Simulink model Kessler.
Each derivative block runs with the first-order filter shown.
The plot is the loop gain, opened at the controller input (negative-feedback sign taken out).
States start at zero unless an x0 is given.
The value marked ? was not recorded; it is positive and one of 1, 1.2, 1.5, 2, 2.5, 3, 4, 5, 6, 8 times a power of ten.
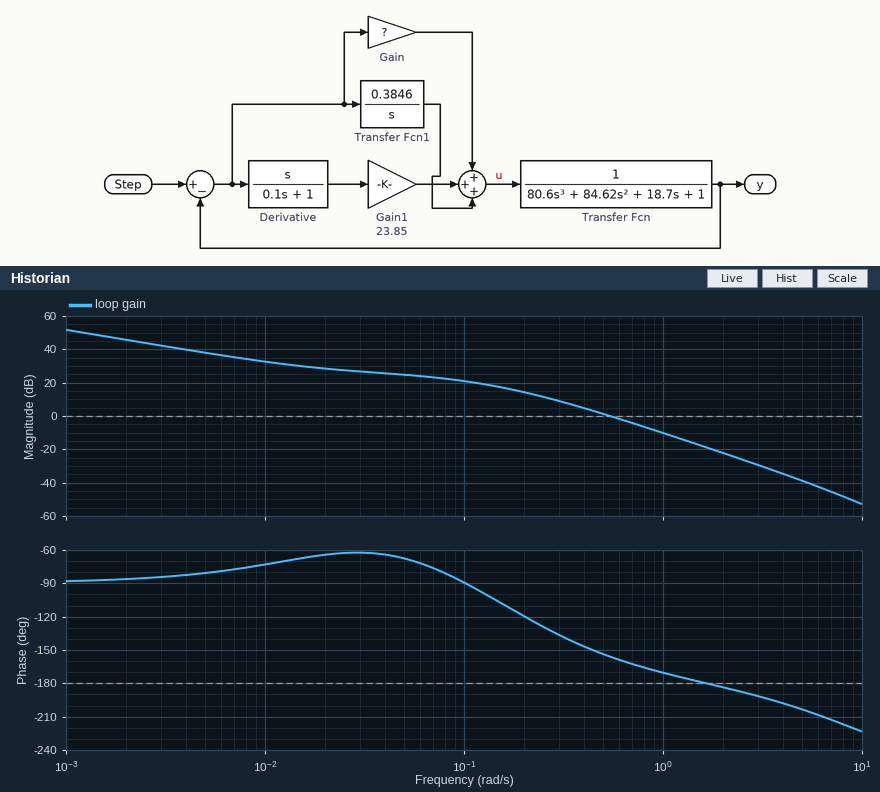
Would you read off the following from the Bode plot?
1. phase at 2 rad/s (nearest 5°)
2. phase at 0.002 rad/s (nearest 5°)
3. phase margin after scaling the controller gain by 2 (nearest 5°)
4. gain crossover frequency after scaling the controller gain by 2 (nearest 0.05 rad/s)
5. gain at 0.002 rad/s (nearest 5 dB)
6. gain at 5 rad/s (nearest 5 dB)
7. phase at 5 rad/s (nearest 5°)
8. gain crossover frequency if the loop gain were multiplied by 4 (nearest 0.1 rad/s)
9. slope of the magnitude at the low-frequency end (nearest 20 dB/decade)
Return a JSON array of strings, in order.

["-185°", "-85°", "15°", "0.80 rad/s", "45 dB", "-40 dB", "-205°", "1.1 rad/s", "-20 dB/decade"]
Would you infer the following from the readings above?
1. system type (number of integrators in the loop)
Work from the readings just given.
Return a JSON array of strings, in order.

["1"]
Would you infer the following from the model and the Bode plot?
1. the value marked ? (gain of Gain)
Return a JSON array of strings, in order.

["20"]
